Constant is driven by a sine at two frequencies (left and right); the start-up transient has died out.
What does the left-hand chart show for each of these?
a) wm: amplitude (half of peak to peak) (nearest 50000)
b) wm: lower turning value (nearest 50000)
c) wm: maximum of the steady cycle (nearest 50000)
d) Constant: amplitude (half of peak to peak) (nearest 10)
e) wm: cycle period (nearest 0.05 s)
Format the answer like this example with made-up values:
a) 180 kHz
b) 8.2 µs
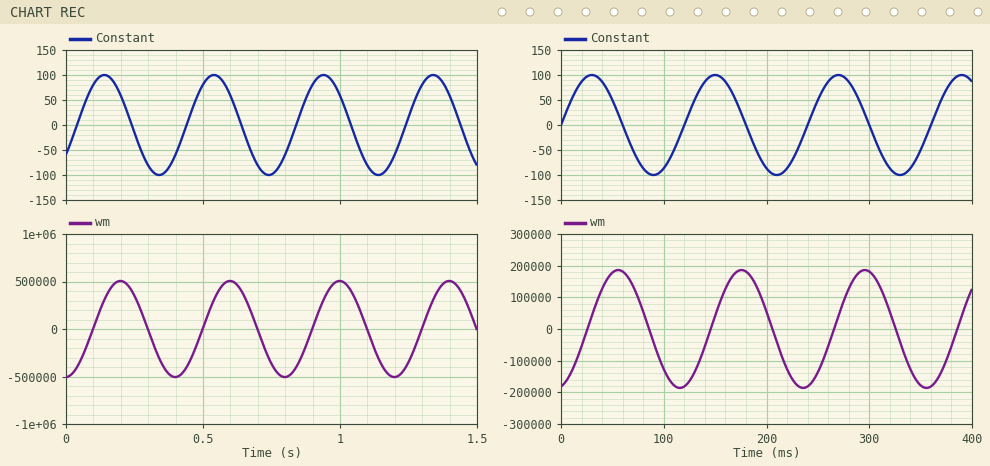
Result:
a) 500000
b) -500000
c) 500000
d) 100
e) 0.40 s
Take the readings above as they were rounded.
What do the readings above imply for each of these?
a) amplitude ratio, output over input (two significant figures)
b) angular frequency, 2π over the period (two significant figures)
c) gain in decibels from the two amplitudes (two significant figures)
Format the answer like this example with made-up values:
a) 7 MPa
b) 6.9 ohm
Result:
a) 5000
b) 16 rad/s
c) 74 dB
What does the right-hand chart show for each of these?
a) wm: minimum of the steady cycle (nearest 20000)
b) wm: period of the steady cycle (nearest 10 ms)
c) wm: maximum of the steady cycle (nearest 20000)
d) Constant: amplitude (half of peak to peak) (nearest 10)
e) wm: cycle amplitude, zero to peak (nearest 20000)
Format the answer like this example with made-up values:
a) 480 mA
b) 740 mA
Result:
a) -180000
b) 120 ms
c) 180000
d) 100
e) 180000
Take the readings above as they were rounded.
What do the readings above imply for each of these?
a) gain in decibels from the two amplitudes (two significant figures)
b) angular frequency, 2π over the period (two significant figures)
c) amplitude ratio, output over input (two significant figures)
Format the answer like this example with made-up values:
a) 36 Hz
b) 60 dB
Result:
a) 65 dB
b) 0.052 rad/ms
c) 1800
